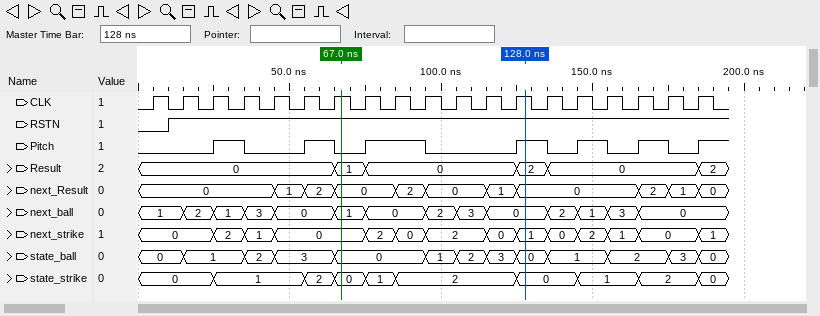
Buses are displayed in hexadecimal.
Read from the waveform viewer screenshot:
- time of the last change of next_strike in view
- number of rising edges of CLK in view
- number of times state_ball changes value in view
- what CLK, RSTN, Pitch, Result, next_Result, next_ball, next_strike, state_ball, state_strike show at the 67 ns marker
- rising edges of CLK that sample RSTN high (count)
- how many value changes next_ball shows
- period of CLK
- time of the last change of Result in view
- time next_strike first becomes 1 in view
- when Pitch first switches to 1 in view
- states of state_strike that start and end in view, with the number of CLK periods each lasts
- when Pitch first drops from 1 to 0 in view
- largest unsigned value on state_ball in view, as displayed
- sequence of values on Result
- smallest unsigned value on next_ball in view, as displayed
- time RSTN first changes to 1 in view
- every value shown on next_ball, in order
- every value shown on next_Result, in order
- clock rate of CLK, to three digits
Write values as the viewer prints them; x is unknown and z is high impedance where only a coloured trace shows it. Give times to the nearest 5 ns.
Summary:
185 ns
19
12
CLK=1, RSTN=1, Pitch=0, Result=1, next_Result=0, next_ball=1, next_strike=0, state_ball=0, state_strike=0
18
13
10 ns
185 ns
35 ns
25 ns
1: 3, 2: 1, 0: 1, 1: 1, 2: 4, 0: 2, 1: 2, 2: 2
35 ns
3
0, 1, 0, 2, 0, 2
0
10 ns
1, 2, 1, 3, 0, 1, 0, 2, 3, 0, 2, 1, 3, 0
0, 1, 2, 0, 2, 0, 1, 0, 2, 1, 0
100 MHz
